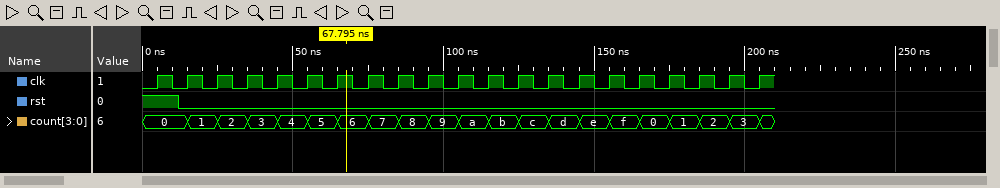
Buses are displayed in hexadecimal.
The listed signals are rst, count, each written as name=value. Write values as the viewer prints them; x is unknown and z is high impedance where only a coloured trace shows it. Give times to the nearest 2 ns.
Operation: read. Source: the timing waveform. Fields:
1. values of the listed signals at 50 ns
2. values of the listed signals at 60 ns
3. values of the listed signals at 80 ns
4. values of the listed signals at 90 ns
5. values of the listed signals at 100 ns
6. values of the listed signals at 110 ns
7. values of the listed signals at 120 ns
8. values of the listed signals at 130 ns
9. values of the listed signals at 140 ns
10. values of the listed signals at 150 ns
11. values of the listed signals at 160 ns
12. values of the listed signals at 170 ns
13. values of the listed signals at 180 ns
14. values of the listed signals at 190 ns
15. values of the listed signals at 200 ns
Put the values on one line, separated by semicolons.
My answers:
rst=0, count=4; rst=0, count=5; rst=0, count=7; rst=0, count=8; rst=0, count=9; rst=0, count=a; rst=0, count=b; rst=0, count=c; rst=0, count=d; rst=0, count=e; rst=0, count=f; rst=0, count=0; rst=0, count=1; rst=0, count=2; rst=0, count=3
